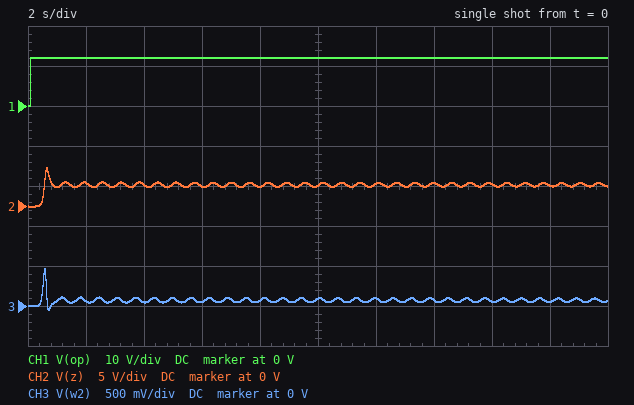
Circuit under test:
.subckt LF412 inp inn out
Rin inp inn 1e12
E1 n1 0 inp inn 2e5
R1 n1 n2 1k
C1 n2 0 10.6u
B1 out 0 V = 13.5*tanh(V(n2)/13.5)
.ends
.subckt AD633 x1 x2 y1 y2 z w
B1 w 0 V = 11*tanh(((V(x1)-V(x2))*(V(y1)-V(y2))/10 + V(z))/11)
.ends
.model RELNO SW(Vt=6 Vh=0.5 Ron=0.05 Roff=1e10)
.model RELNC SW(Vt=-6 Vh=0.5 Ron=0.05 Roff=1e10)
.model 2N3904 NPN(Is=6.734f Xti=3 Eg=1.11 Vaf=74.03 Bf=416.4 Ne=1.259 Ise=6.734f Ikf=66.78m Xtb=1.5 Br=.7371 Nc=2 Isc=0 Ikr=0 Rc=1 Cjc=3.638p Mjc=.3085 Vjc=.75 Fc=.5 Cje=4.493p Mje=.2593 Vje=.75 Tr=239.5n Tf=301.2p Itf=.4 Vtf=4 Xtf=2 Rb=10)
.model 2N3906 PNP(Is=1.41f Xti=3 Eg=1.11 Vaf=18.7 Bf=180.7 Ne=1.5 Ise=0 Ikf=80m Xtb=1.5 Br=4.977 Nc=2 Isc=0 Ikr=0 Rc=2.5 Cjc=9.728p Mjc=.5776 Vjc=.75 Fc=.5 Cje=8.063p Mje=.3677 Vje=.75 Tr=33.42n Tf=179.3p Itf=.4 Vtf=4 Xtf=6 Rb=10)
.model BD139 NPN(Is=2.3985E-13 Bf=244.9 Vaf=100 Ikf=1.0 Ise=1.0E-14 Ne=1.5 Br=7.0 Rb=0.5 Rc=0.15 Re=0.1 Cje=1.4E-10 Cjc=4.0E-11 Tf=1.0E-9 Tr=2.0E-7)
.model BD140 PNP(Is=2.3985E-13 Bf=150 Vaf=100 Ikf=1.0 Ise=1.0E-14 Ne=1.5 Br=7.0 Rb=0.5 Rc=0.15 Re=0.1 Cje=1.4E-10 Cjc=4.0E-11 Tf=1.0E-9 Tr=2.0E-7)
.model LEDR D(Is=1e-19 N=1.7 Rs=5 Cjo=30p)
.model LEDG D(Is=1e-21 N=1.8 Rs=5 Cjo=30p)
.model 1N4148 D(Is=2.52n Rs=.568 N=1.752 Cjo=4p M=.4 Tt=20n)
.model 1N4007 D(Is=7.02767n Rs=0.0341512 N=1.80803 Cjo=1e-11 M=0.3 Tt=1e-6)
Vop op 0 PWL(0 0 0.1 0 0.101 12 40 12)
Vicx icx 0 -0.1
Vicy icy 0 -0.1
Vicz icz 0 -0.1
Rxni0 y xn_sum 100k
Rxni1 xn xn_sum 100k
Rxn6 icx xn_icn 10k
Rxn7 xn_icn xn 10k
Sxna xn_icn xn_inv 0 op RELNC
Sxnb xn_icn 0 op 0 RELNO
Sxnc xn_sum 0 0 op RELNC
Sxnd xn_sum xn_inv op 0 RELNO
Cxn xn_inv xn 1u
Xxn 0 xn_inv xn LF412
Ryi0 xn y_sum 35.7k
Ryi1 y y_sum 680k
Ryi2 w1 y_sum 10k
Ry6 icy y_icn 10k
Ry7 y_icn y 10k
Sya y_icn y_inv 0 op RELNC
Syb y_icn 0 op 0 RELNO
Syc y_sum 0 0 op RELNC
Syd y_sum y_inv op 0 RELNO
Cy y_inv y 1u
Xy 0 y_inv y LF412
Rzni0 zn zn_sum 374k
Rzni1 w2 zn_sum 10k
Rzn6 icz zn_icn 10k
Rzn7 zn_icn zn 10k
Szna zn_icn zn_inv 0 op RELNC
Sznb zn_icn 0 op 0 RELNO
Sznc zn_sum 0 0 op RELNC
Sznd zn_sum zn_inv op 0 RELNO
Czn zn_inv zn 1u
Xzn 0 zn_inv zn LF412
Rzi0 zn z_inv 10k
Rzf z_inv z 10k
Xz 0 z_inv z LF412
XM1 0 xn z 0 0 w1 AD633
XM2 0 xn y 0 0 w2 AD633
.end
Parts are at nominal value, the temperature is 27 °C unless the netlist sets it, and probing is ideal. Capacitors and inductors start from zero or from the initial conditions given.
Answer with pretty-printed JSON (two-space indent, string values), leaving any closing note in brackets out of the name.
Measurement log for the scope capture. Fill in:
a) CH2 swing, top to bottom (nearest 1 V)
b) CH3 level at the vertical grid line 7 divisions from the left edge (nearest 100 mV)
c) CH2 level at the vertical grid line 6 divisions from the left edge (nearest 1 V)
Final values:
{
  "CH2 swing, top to bottom": "5 V",
  "CH3 level at the vertical grid line 7 divisions from the left edge": "100 mV",
  "CH2 level at the vertical grid line 6 divisions from the left edge": "3 V"
}
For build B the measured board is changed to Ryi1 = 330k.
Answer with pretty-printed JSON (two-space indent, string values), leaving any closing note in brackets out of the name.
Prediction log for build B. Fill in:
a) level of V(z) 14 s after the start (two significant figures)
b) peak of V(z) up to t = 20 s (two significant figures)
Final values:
{
  "level of V(z) 14 s after the start": "2.5 V",
  "peak of V(z) up to t = 20 s": "4.3 V"
}
